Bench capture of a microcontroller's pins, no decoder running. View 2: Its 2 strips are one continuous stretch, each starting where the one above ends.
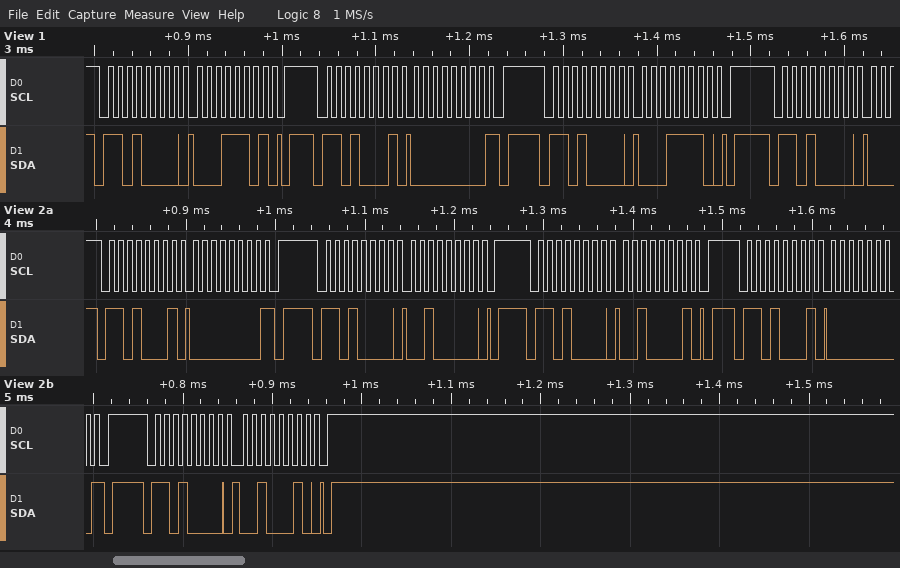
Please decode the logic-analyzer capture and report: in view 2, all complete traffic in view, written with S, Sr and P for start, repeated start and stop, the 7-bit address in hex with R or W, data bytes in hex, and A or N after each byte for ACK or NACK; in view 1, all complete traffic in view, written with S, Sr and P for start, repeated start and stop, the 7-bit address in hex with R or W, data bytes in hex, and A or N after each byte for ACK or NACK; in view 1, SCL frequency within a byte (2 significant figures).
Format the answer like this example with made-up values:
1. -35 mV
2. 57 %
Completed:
1. S 68R A 00 N P S 68W A 20 A P S 68W A 21 A P S 68R A 00 N P S 68W A 22 A P
2. S 68W A 1D A P S 68R A 00 N P S 68W A 1E A P S 68W A
3. 100 kHz
